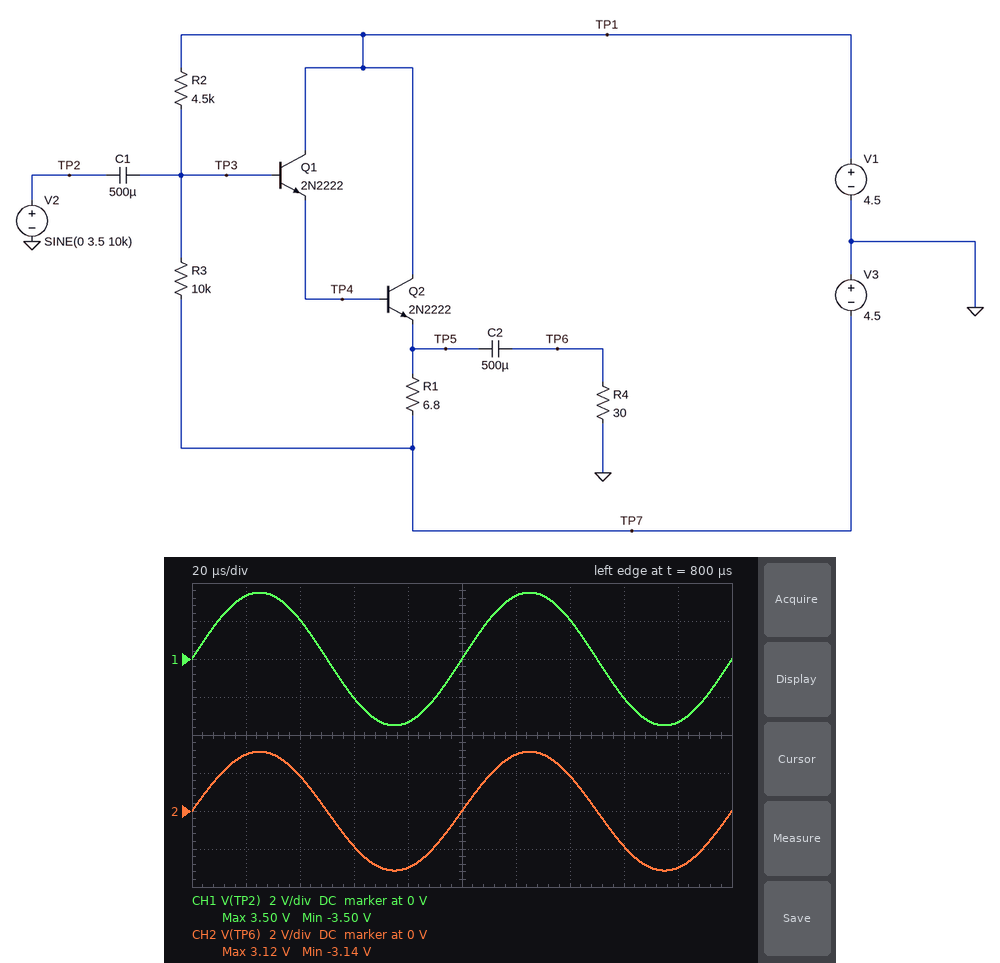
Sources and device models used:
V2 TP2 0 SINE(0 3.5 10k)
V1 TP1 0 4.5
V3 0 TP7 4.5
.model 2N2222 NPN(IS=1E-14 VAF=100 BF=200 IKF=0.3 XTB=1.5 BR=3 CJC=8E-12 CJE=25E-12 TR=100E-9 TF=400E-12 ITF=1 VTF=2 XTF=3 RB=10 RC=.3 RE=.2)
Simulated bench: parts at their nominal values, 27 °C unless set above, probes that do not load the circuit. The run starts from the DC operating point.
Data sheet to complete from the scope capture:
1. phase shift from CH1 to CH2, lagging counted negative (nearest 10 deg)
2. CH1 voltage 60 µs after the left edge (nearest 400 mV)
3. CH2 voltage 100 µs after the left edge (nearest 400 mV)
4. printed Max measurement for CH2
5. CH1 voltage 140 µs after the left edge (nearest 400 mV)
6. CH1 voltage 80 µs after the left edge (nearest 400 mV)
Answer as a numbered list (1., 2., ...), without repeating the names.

1. 0 deg
2. -2.0 V
3. 0 V
4. 3.12 V
5. 2.0 V
6. -3.2 V
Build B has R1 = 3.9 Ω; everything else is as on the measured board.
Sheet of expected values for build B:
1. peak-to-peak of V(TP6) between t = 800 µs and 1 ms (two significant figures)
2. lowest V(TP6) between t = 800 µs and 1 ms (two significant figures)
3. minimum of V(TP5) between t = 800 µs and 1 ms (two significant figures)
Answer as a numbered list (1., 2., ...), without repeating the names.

1. 5.8 V
2. -3.0 V
3. -3.6 V
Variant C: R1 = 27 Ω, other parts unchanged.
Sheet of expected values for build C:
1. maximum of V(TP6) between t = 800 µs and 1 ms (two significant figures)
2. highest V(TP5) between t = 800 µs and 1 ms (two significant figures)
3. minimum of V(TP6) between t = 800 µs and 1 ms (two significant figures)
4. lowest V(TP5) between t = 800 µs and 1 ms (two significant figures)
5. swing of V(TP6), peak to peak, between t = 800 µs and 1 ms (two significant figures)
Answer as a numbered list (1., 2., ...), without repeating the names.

1. 3.3 V
2. 3.5 V
3. -2.5 V
4. -2.3 V
5. 5.8 V
